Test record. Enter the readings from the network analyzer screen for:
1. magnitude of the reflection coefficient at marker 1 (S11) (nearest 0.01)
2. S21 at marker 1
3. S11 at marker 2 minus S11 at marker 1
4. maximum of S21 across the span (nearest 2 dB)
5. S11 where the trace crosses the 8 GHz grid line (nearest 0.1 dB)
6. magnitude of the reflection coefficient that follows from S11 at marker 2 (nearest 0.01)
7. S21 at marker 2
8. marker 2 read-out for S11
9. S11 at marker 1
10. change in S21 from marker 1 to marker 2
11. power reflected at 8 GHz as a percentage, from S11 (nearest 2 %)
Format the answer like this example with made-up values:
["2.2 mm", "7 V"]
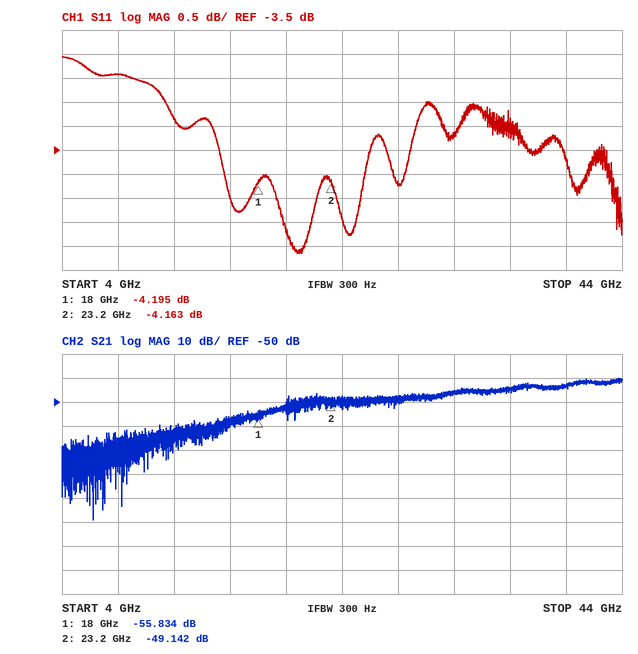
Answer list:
["0.62", "-55.834 dB", "0.032 dB", "-40 dB", "-1.9 dB", "0.62", "-49.142 dB", "-4.163 dB", "-4.195 dB", "6.692 dB", "64 %"]
